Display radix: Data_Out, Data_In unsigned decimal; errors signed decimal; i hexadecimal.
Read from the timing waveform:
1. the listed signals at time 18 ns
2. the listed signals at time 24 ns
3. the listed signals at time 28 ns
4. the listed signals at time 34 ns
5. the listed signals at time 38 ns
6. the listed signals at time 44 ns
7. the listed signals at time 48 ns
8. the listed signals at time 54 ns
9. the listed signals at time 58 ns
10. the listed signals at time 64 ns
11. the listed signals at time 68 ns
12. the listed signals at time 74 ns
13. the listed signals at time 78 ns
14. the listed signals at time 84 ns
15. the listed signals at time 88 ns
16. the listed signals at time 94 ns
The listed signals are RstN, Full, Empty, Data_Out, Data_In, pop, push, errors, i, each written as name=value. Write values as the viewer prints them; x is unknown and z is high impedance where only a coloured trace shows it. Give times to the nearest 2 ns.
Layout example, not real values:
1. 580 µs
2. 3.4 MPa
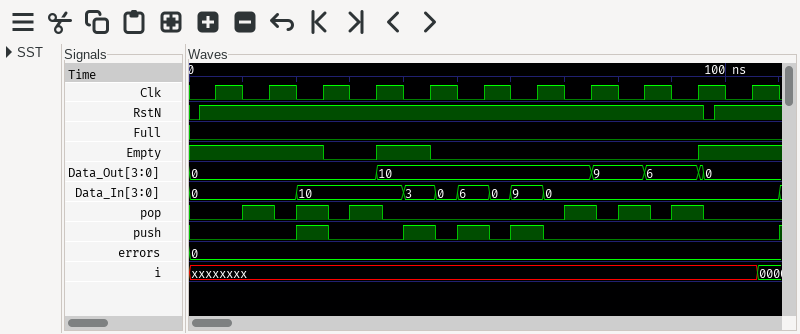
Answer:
1. RstN=1, Full=0, Empty=1, Data_Out=0, Data_In=0, pop=0, push=0, errors=0, i=xxxxxxxx
2. RstN=1, Full=0, Empty=1, Data_Out=0, Data_In=10, pop=1, push=1, errors=0, i=xxxxxxxx
3. RstN=1, Full=0, Empty=0, Data_Out=0, Data_In=10, pop=0, push=0, errors=0, i=xxxxxxxx
4. RstN=1, Full=0, Empty=0, Data_Out=0, Data_In=10, pop=1, push=0, errors=0, i=xxxxxxxx
5. RstN=1, Full=0, Empty=1, Data_Out=10, Data_In=10, pop=0, push=0, errors=0, i=xxxxxxxx
6. RstN=1, Full=0, Empty=1, Data_Out=10, Data_In=3, pop=0, push=1, errors=0, i=xxxxxxxx
7. RstN=1, Full=0, Empty=0, Data_Out=10, Data_In=0, pop=0, push=0, errors=0, i=xxxxxxxx
8. RstN=1, Full=0, Empty=0, Data_Out=10, Data_In=6, pop=0, push=1, errors=0, i=xxxxxxxx
9. RstN=1, Full=0, Empty=0, Data_Out=10, Data_In=0, pop=0, push=0, errors=0, i=xxxxxxxx
10. RstN=1, Full=0, Empty=0, Data_Out=10, Data_In=9, pop=0, push=1, errors=0, i=xxxxxxxx
11. RstN=1, Full=0, Empty=0, Data_Out=10, Data_In=0, pop=0, push=0, errors=0, i=xxxxxxxx
12. RstN=1, Full=0, Empty=0, Data_Out=10, Data_In=0, pop=1, push=0, errors=0, i=xxxxxxxx
13. RstN=1, Full=0, Empty=0, Data_Out=9, Data_In=0, pop=0, push=0, errors=0, i=xxxxxxxx
14. RstN=1, Full=0, Empty=0, Data_Out=9, Data_In=0, pop=1, push=0, errors=0, i=xxxxxxxx
15. RstN=1, Full=0, Empty=0, Data_Out=6, Data_In=0, pop=0, push=0, errors=0, i=xxxxxxxx
16. RstN=1, Full=0, Empty=0, Data_Out=6, Data_In=0, pop=1, push=0, errors=0, i=xxxxxxxx
